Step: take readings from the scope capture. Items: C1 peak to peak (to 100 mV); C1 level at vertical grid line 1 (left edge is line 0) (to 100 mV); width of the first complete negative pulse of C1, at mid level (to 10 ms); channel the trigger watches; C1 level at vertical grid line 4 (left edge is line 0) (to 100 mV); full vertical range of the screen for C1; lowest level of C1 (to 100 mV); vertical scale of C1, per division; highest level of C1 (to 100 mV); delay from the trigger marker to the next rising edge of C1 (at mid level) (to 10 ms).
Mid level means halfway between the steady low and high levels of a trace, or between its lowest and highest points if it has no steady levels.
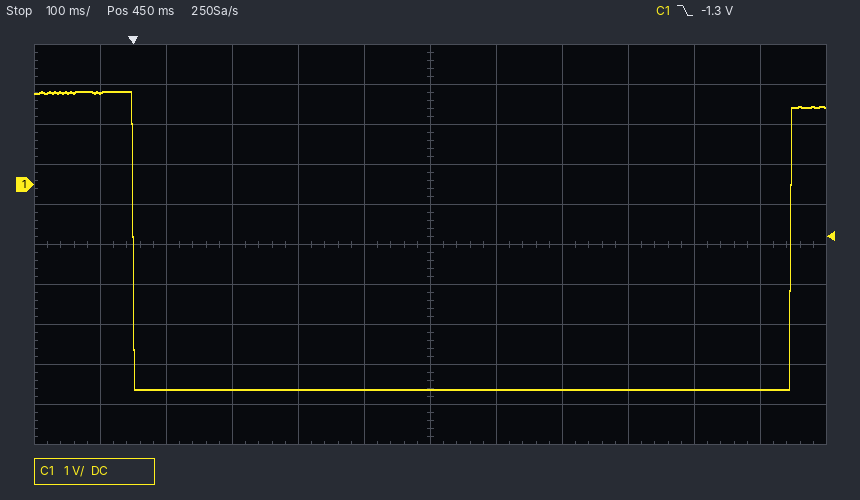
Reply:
7.4 V
2.3 V
1.00 s
C1
-5.1 V
10 V
-5.1 V
1 V
2.3 V
1.00 s
